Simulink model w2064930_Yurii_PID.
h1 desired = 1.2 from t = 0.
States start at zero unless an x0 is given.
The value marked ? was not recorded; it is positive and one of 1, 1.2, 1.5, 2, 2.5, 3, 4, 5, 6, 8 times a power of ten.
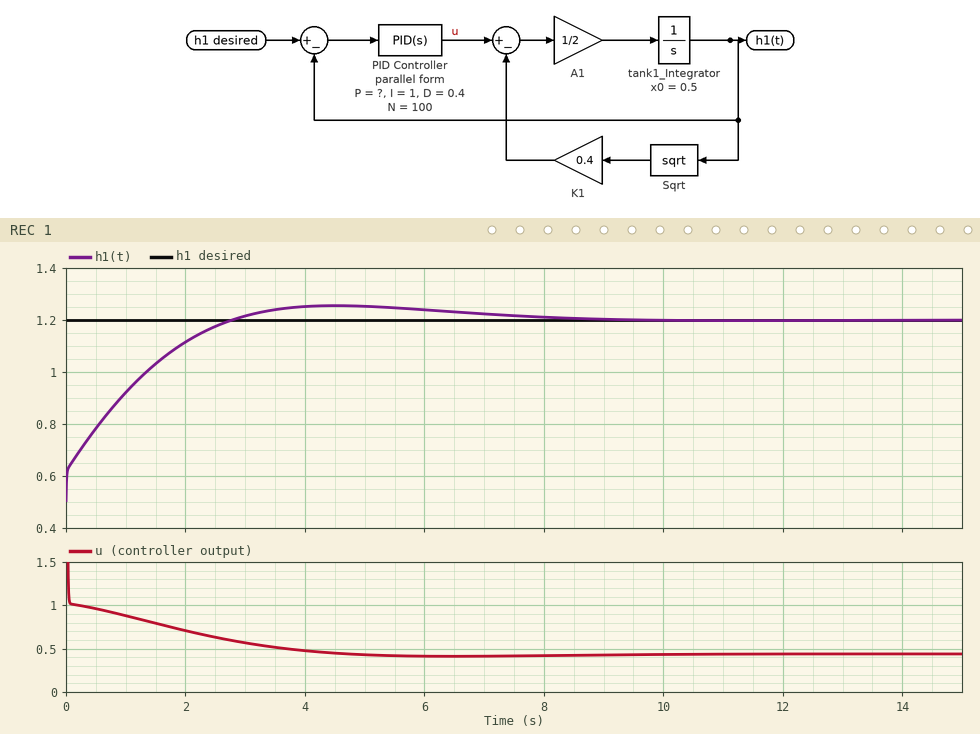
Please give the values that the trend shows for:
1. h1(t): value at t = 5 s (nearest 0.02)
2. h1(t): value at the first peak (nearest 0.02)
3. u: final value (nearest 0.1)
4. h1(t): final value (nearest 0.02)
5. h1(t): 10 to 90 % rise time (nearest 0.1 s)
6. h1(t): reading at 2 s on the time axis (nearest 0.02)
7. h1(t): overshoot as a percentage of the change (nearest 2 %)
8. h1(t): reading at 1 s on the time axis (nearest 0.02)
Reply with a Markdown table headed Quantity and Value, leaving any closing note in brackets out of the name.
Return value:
| Quantity | Value |
|---|---|
| h1(t): value at t = 5 s | 1.26 |
| h1(t): value at the first peak | 1.26 |
| u: final value | 0.4 |
| h1(t): final value | 1.20 |
| h1(t): 10 to 90 % rise time | 2.1 s |
| h1(t): reading at 2 s on the time axis | 1.12 |
| h1(t): overshoot as a percentage of the change | 8 % |
| h1(t): reading at 1 s on the time axis | 0.92 |
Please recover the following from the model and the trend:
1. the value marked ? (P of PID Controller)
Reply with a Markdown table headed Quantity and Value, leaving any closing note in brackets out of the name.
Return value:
| Quantity | Value |
|---|---|
| the value marked ? | 2 |
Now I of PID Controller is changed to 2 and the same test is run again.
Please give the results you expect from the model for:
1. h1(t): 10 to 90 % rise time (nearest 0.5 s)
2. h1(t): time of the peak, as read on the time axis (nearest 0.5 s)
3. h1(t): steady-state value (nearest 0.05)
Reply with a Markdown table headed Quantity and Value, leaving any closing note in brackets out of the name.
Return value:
| Quantity | Value |
|---|---|
| h1(t): 10 to 90 % rise time | 1.5 s |
| h1(t): time of the peak, as read on the time axis | 3.0 s |
| h1(t): steady-state value | 1.20 |
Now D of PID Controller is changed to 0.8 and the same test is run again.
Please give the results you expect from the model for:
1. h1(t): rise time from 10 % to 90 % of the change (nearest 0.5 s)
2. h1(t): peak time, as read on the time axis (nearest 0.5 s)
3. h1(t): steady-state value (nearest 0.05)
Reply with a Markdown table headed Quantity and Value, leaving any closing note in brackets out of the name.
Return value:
| Quantity | Value |
|---|---|
| h1(t): rise time from 10 % to 90 % of the change | 2.5 s |
| h1(t): peak time, as read on the time axis | 5.0 s |
| h1(t): steady-state value | 1.20 |
